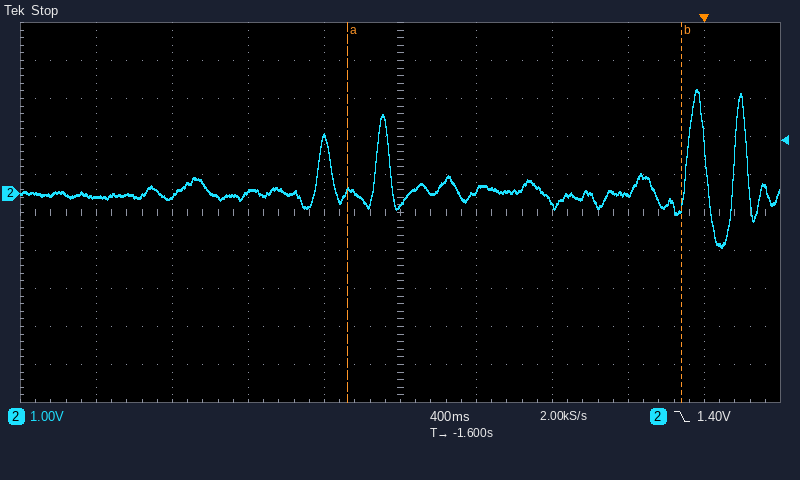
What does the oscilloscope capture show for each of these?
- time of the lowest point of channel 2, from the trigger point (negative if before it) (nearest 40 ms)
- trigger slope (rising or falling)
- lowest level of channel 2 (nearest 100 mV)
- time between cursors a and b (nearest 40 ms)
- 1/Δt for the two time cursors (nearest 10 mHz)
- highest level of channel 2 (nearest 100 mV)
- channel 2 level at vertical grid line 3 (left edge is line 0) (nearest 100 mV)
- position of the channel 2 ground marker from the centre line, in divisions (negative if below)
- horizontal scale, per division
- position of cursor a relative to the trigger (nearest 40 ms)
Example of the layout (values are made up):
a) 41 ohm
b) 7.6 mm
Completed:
a) +80 ms
b) falling
c) -1.4 V
d) 1.76 s
e) 570 mHz
f) 2.7 V
g) 0.0 V
h) +0.5 div
i) 400 ms
j) -1.88 s
